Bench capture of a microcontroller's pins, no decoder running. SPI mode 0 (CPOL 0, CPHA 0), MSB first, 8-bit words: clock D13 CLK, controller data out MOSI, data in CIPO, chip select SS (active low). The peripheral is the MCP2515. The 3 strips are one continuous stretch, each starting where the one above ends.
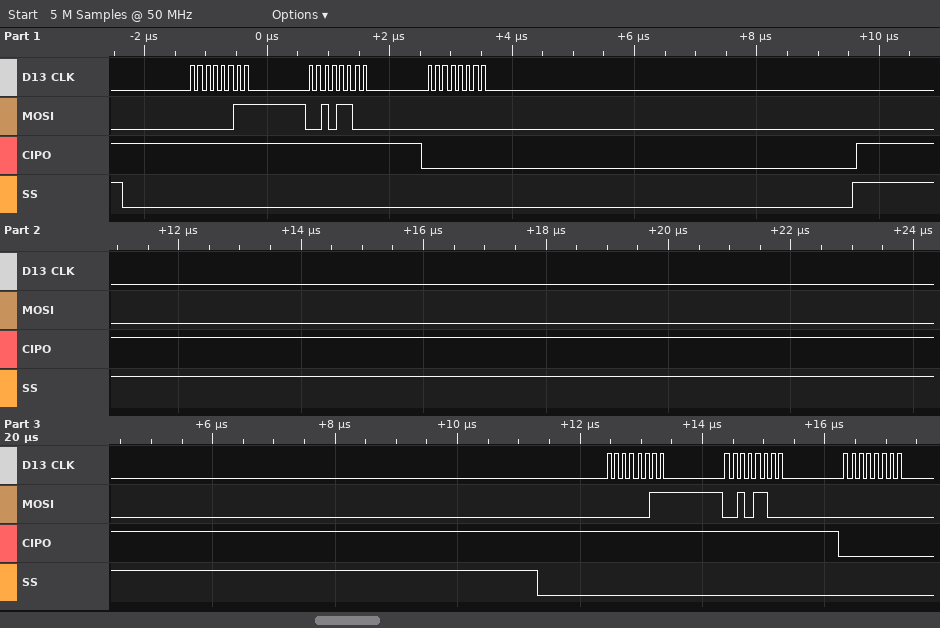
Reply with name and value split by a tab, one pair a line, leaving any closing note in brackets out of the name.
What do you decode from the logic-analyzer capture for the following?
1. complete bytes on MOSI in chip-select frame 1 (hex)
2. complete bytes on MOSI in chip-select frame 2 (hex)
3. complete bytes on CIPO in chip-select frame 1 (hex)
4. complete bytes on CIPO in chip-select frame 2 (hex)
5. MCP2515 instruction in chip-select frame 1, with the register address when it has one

complete bytes on MOSI in chip-select frame 1	03 2C 00
complete bytes on MOSI in chip-select frame 2	03 2C 00
complete bytes on CIPO in chip-select frame 1	FF FF 00
complete bytes on CIPO in chip-select frame 2	FF FF 00
MCP2515 instruction in chip-select frame 1, with the register address when it has one	READ 0x2C
